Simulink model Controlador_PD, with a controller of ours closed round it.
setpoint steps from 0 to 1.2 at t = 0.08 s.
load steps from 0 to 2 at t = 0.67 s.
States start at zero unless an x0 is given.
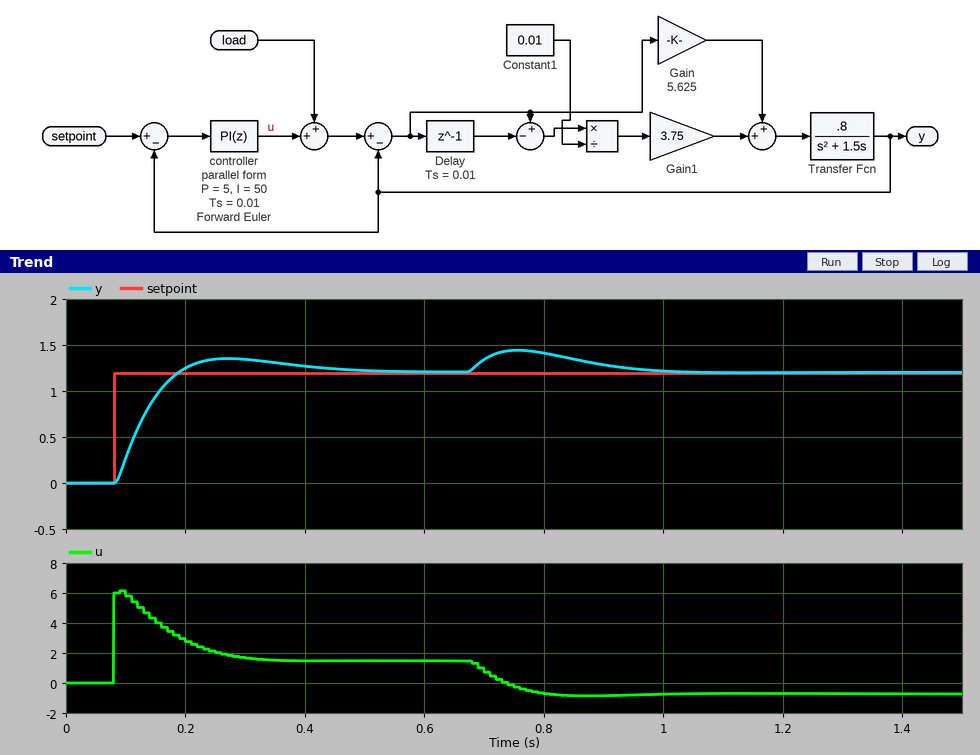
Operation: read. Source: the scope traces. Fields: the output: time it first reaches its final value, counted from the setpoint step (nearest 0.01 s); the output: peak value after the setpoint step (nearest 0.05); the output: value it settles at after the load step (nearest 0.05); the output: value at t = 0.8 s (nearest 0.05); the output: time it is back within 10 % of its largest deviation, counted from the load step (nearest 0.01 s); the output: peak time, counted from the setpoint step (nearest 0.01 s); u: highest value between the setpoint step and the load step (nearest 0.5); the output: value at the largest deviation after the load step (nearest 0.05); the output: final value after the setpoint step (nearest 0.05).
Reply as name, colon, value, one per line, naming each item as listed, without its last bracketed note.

the output: time it first reaches its final value, counted from the setpoint step: 0.11 s
the output: peak value after the setpoint step: 1.35
the output: value it settles at after the load step: 1.20
the output: value at t = 0.8 s: 1.40
the output: time it is back within 10 % of its largest deviation, counted from the load step: 0.31 s
the output: peak time, counted from the setpoint step: 0.19 s
u: highest value between the setpoint step and the load step: 6.0
the output: value at the largest deviation after the load step: 1.45
the output: final value after the setpoint step: 1.20
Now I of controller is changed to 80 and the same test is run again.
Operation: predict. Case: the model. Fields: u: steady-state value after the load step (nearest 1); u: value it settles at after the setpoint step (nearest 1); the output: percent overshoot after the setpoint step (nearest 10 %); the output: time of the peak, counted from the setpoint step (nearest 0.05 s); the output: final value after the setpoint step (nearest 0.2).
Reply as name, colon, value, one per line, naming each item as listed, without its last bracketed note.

u: steady-state value after the load step: -1
u: value it settles at after the setpoint step: 1
the output: percent overshoot after the setpoint step: 20 %
the output: time of the peak, counted from the setpoint step: 0.15 s
the output: final value after the setpoint step: 1.2
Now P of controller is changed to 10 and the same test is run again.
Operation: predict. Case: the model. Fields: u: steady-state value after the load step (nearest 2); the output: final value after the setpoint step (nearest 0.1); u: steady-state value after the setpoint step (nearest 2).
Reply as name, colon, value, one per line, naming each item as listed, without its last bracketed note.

u: steady-state value after the load step: 0
the output: final value after the setpoint step: 1.2
u: steady-state value after the setpoint step: 2
